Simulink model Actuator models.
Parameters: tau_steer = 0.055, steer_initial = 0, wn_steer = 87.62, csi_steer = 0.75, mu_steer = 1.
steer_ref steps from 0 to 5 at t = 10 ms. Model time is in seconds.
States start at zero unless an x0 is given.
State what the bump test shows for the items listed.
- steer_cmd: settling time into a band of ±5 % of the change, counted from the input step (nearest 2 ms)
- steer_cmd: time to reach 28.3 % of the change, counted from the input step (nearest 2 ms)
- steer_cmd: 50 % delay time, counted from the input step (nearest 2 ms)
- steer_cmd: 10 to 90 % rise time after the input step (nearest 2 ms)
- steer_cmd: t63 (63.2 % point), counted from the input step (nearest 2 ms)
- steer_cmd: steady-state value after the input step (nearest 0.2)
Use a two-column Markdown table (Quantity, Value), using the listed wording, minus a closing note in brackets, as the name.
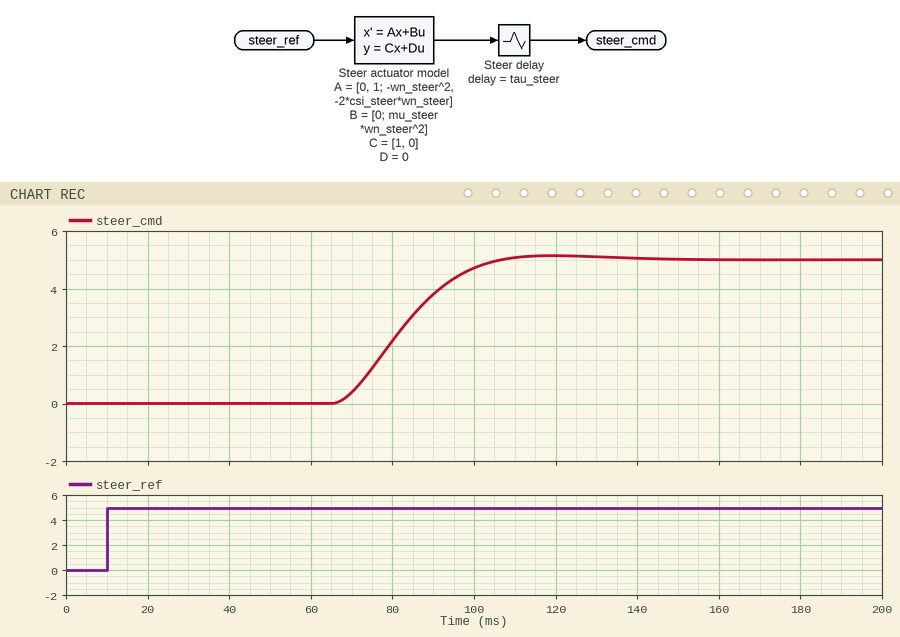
| Quantity | Value |
|---|---|
| steer_cmd: settling time into a band of ±5 % of the change, counted from the input step | 90 ms |
| steer_cmd: time to reach 28.3 % of the change, counted from the input step | 66 ms |
| steer_cmd: 50 % delay time, counted from the input step | 72 ms |
| steer_cmd: 10 to 90 % rise time after the input step | 26 ms |
| steer_cmd: t63 (63.2 % point), counted from the input step | 76 ms |
| steer_cmd: steady-state value after the input step | 5.0 |
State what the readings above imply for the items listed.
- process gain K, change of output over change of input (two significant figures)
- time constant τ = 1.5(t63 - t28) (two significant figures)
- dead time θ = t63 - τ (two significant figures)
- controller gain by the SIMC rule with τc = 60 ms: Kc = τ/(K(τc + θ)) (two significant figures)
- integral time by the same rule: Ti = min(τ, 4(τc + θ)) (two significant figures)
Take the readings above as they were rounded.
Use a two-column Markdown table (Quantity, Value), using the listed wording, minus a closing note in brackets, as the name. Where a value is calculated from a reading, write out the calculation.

| Quantity | Value |
|---|---|
| process gain K, change of output over change of input | (5 - 0) / 5 = 1.0 |
| time constant τ = 1.5(t63 - t28) | 1.5 × (76 - 66) = 15 ms |
| dead time θ = t63 - τ | 76 - 15 = 61 ms |
| controller gain by the SIMC rule with τc = 60 ms: Kc = τ/(K(τc + θ)) | 15 / (1 × (60 + 61)) = 0.12 |
| integral time by the same rule: Ti = min(τ, 4(τc + θ)) | min(15, 4 × (60 + 61)) = 15 ms |
